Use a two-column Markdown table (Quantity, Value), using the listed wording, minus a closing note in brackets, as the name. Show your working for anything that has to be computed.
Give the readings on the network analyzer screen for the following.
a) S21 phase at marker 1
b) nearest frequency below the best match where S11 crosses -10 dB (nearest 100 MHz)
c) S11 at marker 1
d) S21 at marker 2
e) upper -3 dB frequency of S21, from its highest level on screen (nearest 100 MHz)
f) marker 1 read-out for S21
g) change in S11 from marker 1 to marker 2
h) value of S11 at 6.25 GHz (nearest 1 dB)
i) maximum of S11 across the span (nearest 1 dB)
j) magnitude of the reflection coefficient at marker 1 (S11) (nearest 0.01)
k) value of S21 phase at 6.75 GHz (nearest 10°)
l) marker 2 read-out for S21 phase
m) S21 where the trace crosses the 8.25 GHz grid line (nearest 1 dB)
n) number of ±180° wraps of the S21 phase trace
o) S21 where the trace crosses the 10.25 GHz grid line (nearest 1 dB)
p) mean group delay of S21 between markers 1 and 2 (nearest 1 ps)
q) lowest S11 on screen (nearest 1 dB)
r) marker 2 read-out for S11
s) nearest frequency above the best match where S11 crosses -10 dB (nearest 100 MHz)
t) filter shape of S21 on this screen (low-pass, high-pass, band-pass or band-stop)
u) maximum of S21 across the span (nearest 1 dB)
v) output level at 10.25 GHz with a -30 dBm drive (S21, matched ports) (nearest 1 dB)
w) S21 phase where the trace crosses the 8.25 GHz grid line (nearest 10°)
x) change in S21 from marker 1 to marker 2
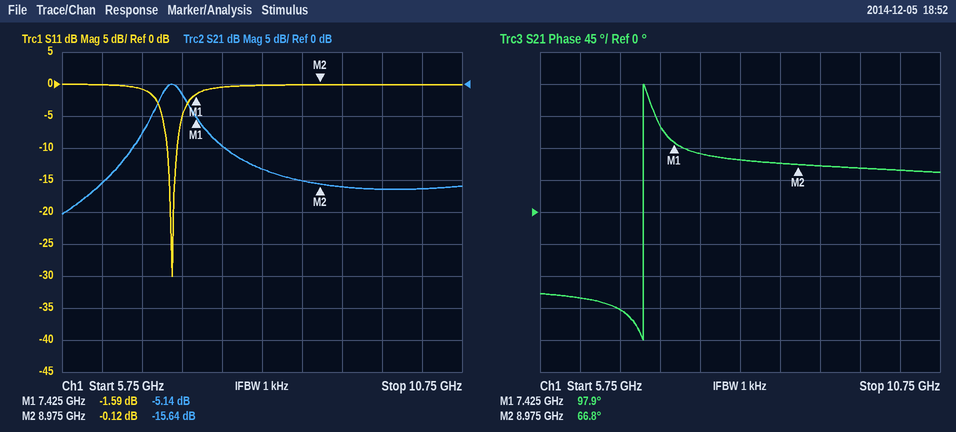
| Quantity | Value |
|---|---|
| S21 phase at marker 1 | 97.9° |
| nearest frequency below the best match where S11 crosses -10 dB | 7.1 GHz |
| S11 at marker 1 | -1.59 dB |
| S21 at marker 2 | -15.64 dB |
| upper -3 dB frequency of S21, from its highest level on screen | 7.3 GHz |
| marker 1 read-out for S21 | -5.14 dB |
| change in S11 from marker 1 to marker 2 | -0.12 − (-1.59) = 1.47 dB |
| value of S11 at 6.25 GHz | 0 dB |
| maximum of S11 across the span | 0 dB |
| magnitude of the reflection coefficient at marker 1 (S11) | 10^(-1.59/20) ≈ 0.83 |
| value of S21 phase at 6.75 GHz | -140° |
| marker 2 read-out for S21 phase | 66.8° |
| S21 where the trace crosses the 8.25 GHz grid line | -13 dB |
| number of ±180° wraps of the S21 phase trace | 1 |
| S21 where the trace crosses the 10.25 GHz grid line | -16 dB |
| mean group delay of S21 between markers 1 and 2 | −(66.8° − (97.9°))/(360° × 1.55 GHz) ≈ 56 ps |
| lowest S11 on screen | -30 dB |
| marker 2 read-out for S11 | -0.12 dB |
| nearest frequency above the best match where S11 crosses -10 dB | 7.2 GHz |
| filter shape of S21 on this screen | band-pass |
| maximum of S21 across the span | 0 dB |
| output level at 10.25 GHz with a -30 dBm drive (S21, matched ports) | -30 dBm + (-16 dB) = -46 dBm |
| S21 phase where the trace crosses the 8.25 GHz grid line | 70° |
| change in S21 from marker 1 to marker 2 | -15.64 − (-5.14) = -10.50 dB |
